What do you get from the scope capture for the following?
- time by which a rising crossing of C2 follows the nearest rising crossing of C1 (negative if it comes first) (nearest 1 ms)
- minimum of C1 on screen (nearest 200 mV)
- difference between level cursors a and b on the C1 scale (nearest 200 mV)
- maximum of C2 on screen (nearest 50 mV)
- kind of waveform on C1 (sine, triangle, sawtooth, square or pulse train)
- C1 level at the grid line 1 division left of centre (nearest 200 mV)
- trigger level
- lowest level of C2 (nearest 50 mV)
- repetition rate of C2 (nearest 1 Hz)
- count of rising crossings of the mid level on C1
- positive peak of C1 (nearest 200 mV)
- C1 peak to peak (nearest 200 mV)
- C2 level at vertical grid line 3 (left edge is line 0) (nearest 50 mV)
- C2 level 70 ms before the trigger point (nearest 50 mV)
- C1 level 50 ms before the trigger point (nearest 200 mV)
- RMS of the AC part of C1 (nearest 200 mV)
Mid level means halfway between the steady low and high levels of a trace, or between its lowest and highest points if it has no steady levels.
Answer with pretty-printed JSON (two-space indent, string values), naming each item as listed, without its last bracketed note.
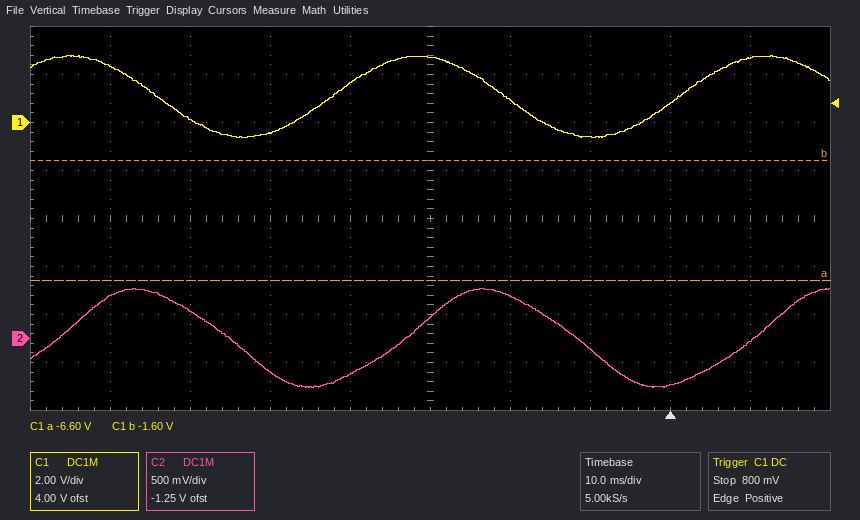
{
  "time by which a rising crossing of C2 follows the nearest rising crossing of C1 (negative if it comes first)": "+9 ms",
  "minimum of C1 on screen": "-600 mV",
  "difference between level cursors a and b on the C1 scale": "5.0 V",
  "maximum of C2 on screen": "500 mV",
  "kind of waveform on C1": "sine",
  "C1 level at the grid line 1 division left of centre": "1.6 V",
  "trigger level": "800 mV",
  "lowest level of C2": "-500 mV",
  "repetition rate of C2": "23 Hz",
  "count of rising crossings of the mid level on C1": "2",
  "positive peak of C1": "2.8 V",
  "C1 peak to peak": "3.4 V",
  "C2 level at vertical grid line 3 (left edge is line 0)": "-350 mV",
  "C2 level 70 ms before the trigger point": "450 mV",
  "C1 level 50 ms before the trigger point": "-400 mV",
  "RMS of the AC part of C1": "1.2 V"
}
